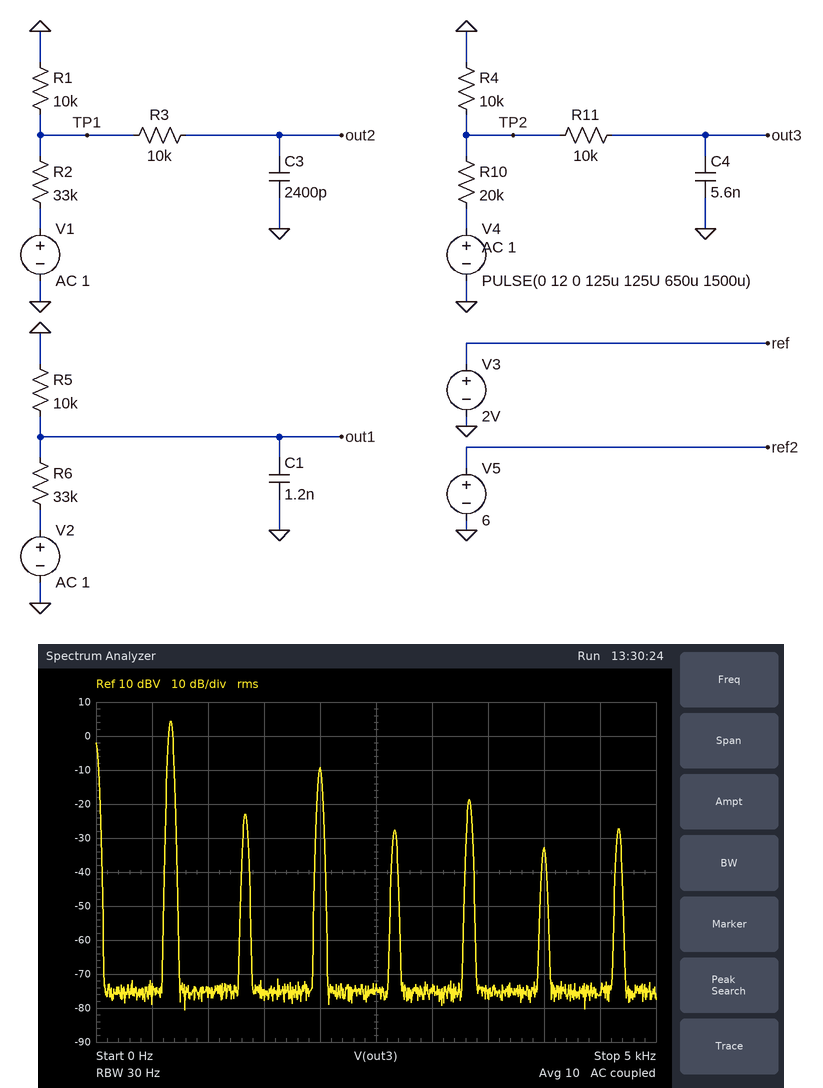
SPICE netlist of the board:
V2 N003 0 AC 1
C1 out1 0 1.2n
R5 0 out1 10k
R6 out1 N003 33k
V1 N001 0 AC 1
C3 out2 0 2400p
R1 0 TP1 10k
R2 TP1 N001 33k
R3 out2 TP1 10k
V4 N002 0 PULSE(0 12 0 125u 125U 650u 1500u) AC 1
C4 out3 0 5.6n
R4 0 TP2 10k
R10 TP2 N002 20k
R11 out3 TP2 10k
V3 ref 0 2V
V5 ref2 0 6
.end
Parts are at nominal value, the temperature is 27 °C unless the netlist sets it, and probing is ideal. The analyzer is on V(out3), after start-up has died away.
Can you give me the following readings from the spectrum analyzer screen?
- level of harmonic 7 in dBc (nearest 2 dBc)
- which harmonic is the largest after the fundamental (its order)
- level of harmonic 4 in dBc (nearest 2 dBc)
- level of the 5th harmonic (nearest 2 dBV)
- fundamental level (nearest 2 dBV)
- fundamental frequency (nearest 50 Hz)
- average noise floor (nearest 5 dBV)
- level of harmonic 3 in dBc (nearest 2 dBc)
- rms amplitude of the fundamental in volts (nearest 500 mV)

-32 dBc
3
-32 dBc
-18 dBV
4 dBV
650 Hz
-75 dBV
-14 dBc
1.5 V
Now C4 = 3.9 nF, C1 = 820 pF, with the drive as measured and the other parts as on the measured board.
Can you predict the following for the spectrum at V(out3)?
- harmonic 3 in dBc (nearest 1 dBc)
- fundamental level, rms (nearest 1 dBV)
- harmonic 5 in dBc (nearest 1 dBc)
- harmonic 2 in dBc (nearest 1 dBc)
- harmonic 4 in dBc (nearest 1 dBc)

-12 dBc
5 dBV
-21 dBc
-27 dBc
-30 dBc
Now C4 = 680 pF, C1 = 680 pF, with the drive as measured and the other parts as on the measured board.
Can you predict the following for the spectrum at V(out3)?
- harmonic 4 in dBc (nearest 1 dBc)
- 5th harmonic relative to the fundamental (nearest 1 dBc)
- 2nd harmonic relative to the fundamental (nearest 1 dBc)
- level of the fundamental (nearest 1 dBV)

-27 dBc
-17 dBc
-26 dBc
5 dBV
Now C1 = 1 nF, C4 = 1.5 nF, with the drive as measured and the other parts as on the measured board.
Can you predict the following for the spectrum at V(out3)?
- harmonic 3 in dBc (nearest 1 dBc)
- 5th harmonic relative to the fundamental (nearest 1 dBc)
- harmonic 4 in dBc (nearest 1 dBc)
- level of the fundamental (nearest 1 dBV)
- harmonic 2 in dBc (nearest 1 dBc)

-11 dBc
-18 dBc
-28 dBc
5 dBV
-26 dBc
